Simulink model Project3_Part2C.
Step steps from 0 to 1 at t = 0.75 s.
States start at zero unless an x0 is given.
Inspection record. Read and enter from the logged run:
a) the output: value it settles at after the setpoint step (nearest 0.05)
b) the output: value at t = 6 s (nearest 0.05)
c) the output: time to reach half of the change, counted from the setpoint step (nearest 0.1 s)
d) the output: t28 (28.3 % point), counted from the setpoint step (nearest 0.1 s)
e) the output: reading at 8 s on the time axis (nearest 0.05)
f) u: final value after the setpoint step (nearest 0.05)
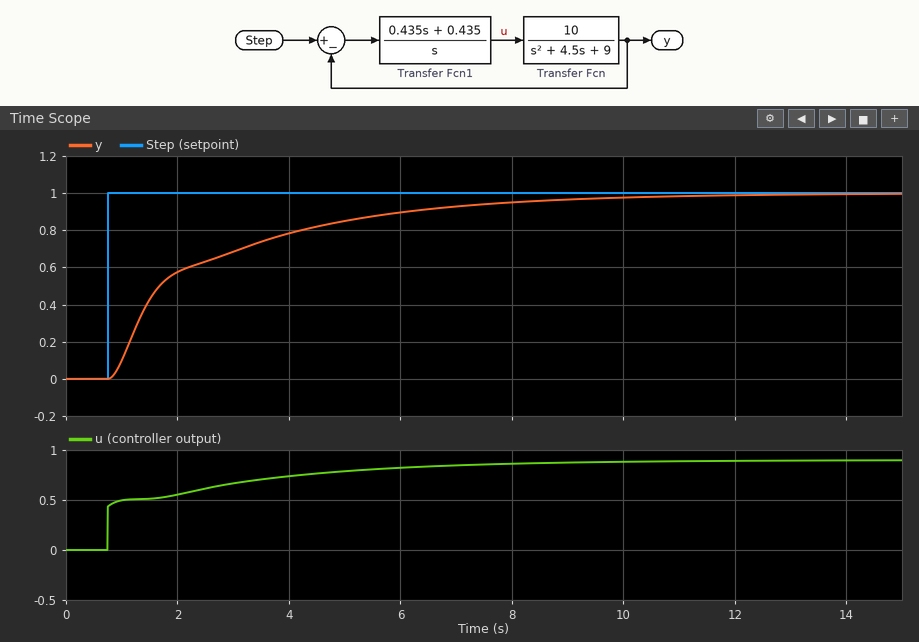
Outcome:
1.00
0.90
0.9 s
0.5 s
0.95
0.90
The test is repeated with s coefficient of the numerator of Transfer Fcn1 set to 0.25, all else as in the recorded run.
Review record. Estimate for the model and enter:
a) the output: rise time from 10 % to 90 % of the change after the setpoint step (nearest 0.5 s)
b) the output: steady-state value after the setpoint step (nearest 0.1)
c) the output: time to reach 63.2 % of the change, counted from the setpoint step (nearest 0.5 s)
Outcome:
4.5 s
1.0
2.0 s
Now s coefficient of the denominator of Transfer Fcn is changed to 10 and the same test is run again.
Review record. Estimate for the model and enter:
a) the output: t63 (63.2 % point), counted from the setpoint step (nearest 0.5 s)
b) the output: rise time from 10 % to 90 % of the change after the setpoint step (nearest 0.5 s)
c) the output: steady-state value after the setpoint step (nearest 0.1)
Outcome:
2.0 s
4.5 s
1.0
